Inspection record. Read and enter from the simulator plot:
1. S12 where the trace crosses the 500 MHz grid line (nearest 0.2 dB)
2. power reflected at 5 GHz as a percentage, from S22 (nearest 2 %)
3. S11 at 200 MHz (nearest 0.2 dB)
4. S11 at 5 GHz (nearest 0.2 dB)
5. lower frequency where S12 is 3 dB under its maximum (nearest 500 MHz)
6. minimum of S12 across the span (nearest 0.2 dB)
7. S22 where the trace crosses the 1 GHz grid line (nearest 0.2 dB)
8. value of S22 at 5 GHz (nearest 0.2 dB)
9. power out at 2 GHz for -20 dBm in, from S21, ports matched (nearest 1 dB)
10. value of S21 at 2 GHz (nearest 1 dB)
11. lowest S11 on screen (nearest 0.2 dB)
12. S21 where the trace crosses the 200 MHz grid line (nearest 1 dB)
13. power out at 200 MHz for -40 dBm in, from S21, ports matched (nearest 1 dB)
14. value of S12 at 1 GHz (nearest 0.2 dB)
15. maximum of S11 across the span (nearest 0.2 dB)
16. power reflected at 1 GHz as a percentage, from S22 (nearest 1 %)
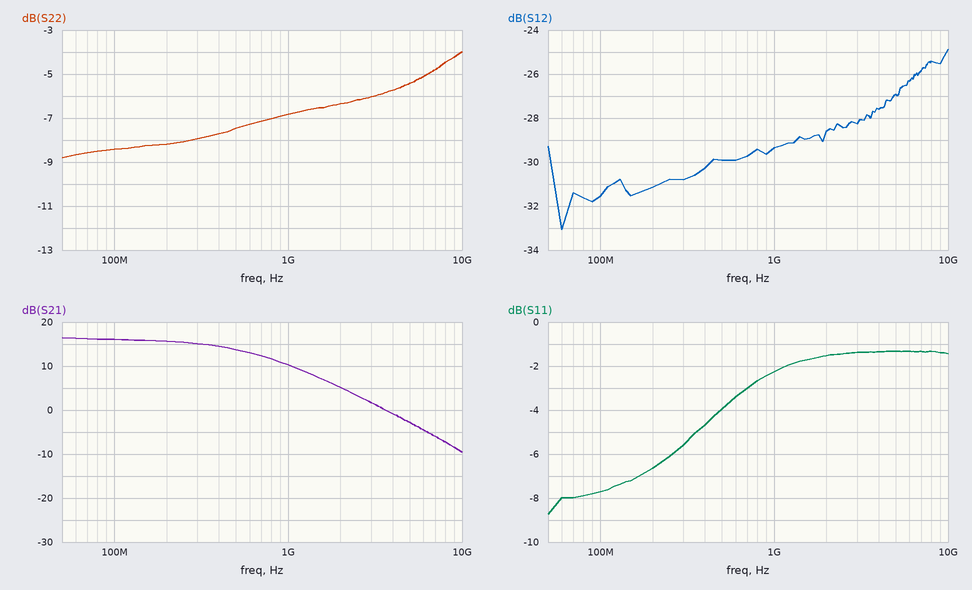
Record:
-30.0 dB
28 %
-6.6 dB
-1.4 dB
3.5 GHz
-33.0 dB
-6.8 dB
-5.4 dB
-15 dBm
5 dB
-8.8 dB
16 dB
-24 dBm
-29.4 dB
-1.4 dB
21 %
